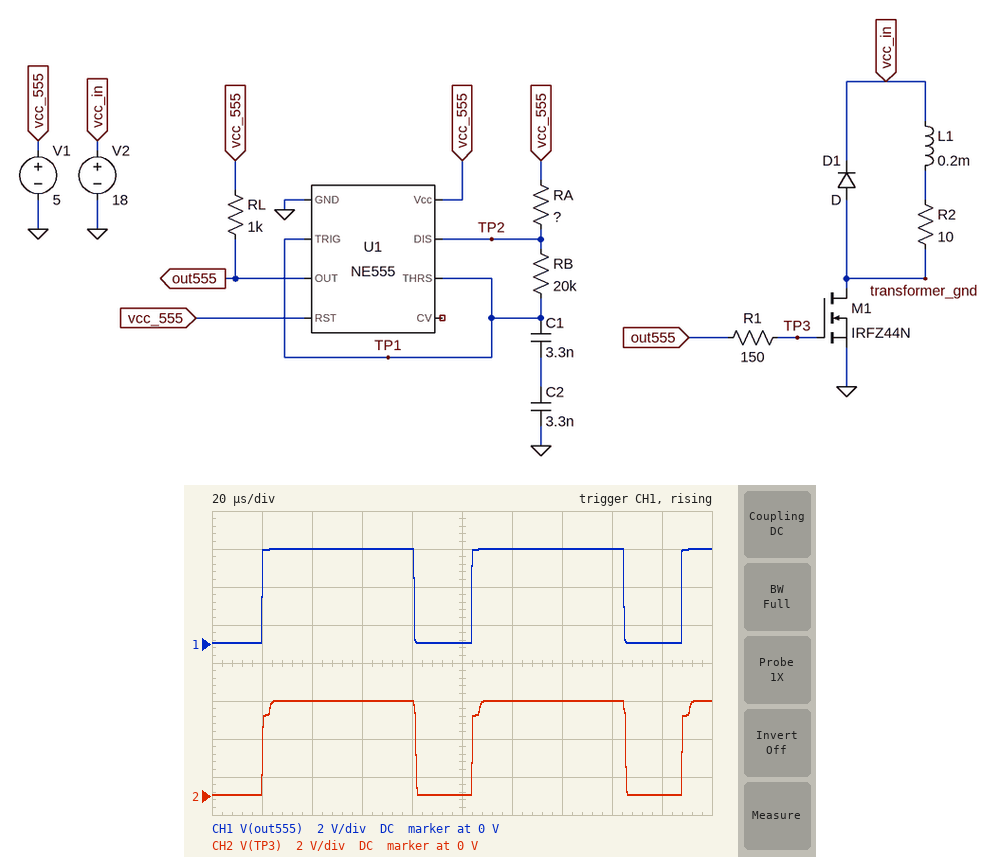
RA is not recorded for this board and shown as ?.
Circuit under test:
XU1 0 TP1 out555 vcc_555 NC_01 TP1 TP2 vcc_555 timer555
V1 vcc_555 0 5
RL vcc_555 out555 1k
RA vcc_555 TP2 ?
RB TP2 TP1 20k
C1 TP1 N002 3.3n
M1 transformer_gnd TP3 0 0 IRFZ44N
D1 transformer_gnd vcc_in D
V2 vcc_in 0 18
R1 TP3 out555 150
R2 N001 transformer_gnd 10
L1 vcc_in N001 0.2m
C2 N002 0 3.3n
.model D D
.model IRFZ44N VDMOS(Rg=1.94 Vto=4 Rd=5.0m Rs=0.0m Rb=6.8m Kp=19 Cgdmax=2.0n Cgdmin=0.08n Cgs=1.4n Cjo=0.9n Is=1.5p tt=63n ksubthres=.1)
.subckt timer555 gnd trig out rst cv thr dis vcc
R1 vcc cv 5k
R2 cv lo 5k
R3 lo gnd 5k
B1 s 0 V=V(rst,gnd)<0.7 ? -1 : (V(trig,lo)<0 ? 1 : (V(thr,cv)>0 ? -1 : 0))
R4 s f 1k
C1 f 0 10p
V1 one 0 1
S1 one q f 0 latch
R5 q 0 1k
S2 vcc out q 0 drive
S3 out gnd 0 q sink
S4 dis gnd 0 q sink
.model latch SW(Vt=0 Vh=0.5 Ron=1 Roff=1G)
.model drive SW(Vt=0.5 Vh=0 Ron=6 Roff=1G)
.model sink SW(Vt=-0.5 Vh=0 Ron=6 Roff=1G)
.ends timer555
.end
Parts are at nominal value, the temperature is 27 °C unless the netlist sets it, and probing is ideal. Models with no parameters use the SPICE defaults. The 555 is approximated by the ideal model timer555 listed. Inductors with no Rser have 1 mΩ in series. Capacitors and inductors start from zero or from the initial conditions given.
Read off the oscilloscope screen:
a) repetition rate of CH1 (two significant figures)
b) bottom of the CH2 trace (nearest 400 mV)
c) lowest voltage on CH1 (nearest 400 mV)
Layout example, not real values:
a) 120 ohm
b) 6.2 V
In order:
a) 12 kHz
b) 0 V
c) 0 V
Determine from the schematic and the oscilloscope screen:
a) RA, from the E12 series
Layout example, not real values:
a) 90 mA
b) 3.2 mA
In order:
a) 33 kΩ
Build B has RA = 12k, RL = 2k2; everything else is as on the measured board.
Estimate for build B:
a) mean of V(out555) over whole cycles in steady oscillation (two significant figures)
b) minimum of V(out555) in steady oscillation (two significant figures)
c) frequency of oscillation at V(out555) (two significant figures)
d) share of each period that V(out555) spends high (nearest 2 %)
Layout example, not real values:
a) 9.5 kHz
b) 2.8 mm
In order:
a) 3.1 V
b) 14 mV
c) 17 kHz
d) 62 %
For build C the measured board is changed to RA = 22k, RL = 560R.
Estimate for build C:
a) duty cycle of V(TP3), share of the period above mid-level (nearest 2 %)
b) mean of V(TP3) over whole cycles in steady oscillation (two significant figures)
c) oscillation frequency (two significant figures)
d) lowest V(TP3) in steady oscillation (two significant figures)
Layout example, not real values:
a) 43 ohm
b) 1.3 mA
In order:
a) 68 %
b) 3.4 V
c) 14 kHz
d) 53 mV
